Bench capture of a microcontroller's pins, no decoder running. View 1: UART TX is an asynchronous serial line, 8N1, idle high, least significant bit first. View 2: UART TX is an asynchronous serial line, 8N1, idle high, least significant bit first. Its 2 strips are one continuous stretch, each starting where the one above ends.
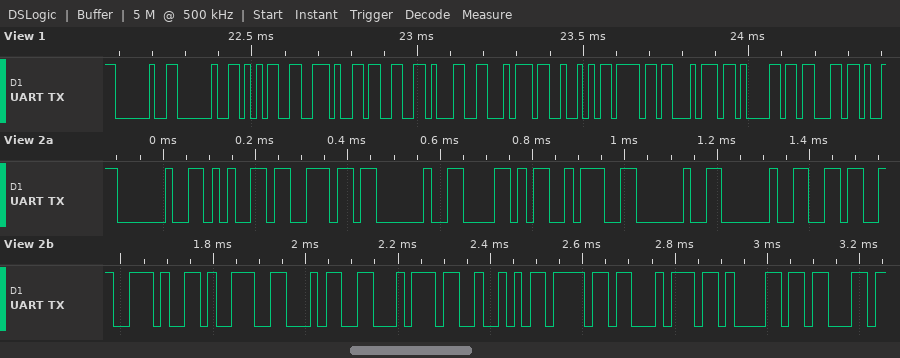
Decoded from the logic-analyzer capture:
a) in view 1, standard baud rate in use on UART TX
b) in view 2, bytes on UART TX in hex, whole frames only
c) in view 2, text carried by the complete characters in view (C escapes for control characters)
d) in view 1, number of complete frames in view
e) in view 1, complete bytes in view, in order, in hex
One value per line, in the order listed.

57600 baud
20 65 6E 20 58 3A 20 20 36 2E 39 34 74 52 6F 74 61 63
" en X:  6.94tRotac"
12
0x20 0x20 0x35 0x2E 0x33 0x31 0x74 0x52 0x6F 0x74 0x61 0x63
